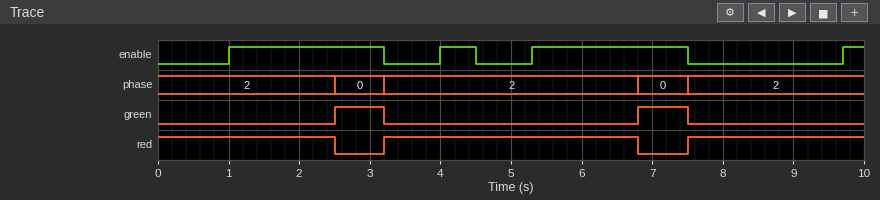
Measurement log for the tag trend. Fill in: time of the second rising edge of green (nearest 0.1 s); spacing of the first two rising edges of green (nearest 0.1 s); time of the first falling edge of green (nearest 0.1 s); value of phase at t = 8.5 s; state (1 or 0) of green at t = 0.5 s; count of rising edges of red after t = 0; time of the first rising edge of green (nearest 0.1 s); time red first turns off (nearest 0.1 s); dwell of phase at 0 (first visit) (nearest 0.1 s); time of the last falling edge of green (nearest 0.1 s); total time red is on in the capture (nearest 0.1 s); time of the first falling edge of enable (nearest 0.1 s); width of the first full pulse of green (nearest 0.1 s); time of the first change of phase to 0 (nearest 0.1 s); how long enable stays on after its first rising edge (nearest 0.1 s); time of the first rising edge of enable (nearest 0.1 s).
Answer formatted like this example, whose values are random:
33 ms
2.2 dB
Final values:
6.8 s
4.3 s
3.2 s
2
0
2
2.5 s
2.5 s
0.7 s
7.5 s
8.6 s
3.2 s
0.7 s
2.5 s
2.2 s
1.0 s
